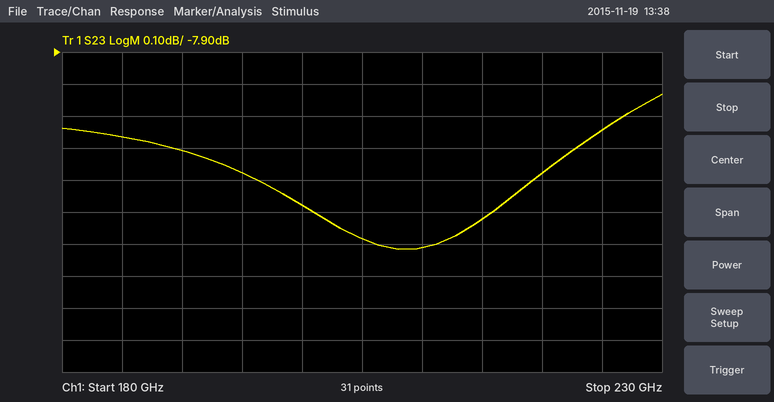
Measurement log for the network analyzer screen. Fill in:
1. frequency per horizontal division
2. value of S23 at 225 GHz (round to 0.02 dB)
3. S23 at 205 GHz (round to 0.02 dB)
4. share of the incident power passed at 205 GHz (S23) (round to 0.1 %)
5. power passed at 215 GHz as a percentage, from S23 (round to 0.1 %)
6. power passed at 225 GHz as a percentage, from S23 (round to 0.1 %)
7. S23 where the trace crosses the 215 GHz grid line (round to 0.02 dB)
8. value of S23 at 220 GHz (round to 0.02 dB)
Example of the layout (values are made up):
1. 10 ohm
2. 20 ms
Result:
1. 5 GHz
2. -8.14 dB
3. -8.48 dB
4. 14.2 %
5. 14.4 %
6. 15.3 %
7. -8.42 dB
8. -8.28 dB
